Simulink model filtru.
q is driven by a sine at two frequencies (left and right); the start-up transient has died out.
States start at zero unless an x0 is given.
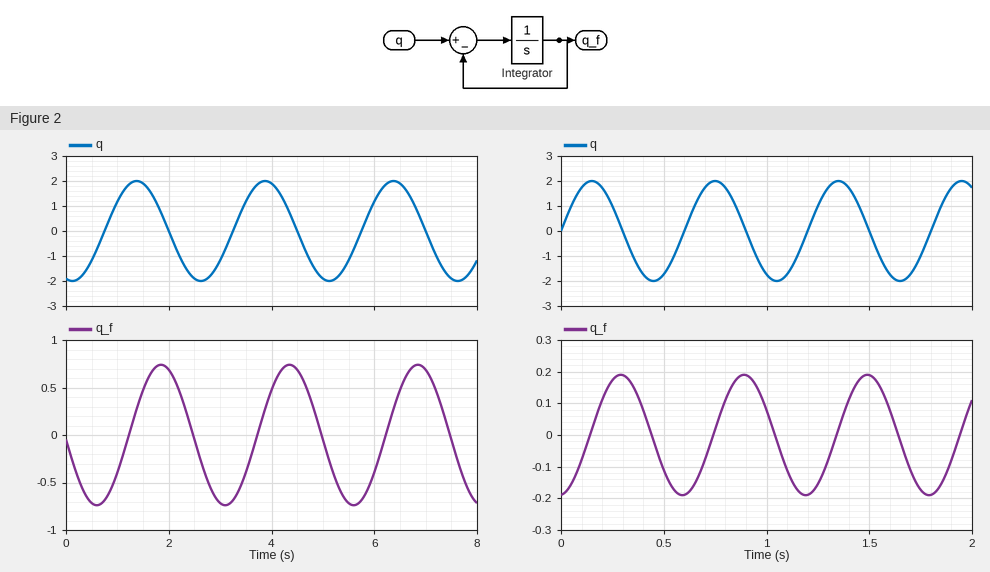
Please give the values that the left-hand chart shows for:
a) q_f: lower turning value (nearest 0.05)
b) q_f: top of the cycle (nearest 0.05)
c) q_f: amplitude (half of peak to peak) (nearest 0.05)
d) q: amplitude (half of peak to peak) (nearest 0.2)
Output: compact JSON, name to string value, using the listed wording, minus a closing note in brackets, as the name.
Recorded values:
{"q_f: lower turning value": "-0.75", "q_f: top of the cycle": "0.75", "q_f: amplitude (half of peak to peak)": "0.75", "q: amplitude (half of peak to peak)": "2.0"}
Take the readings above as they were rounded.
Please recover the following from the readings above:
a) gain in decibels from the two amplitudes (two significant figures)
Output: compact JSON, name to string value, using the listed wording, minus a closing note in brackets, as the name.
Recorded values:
{"gain in decibels from the two amplitudes": "-8.5 dB"}
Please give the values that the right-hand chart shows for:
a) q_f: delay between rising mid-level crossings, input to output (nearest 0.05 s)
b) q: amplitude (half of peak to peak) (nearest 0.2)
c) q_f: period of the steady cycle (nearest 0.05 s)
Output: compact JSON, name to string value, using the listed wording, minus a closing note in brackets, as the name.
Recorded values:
{"q_f: delay between rising mid-level crossings, input to output": "0.15 s", "q: amplitude (half of peak to peak)": "2.0", "q_f: period of the steady cycle": "0.60 s"}
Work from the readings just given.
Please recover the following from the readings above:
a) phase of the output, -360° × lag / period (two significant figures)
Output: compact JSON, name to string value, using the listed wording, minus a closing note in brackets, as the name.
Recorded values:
{"phase of the output, -360° × lag / period": "-90°"}
